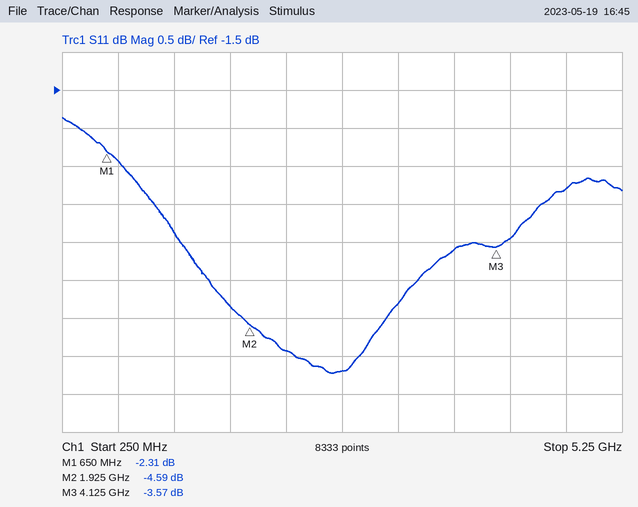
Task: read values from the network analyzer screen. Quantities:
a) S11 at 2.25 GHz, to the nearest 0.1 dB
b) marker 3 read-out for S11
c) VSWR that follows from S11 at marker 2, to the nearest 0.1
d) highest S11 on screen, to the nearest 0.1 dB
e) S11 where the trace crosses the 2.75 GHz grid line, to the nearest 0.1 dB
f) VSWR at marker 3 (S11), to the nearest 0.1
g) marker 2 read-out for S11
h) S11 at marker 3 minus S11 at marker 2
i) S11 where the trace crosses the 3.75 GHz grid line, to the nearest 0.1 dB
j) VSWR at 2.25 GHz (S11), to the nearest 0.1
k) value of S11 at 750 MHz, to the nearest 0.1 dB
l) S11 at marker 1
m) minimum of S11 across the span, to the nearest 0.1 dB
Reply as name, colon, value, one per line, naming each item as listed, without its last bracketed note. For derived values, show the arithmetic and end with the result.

S11 at 2.25 GHz, to the nearest 0.1 dB: -4.9 dB
marker 3 read-out for S11: -3.57 dB
VSWR that follows from S11 at marker 2, to the nearest 0.1: (1 + 0.5895)/(1 − 0.5895) ≈ 3.9
highest S11 on screen, to the nearest 0.1 dB: -1.9 dB
S11 where the trace crosses the 2.75 GHz grid line, to the nearest 0.1 dB: -5.2 dB
VSWR at marker 3 (S11), to the nearest 0.1: (1 + 0.6630)/(1 − 0.6630) ≈ 4.9
marker 2 read-out for S11: -4.59 dB
S11 at marker 3 minus S11 at marker 2: -3.57 − (-4.59) = 1.02 dB
S11 where the trace crosses the 3.75 GHz grid line, to the nearest 0.1 dB: -3.6 dB
VSWR at 2.25 GHz (S11), to the nearest 0.1: |Γ| = 10^(-4.9/20) = 0.5689; VSWR = (1 + 0.5689)/(1 − 0.5689) ≈ 3.6
value of S11 at 750 MHz, to the nearest 0.1 dB: -2.4 dB
S11 at marker 1: -2.31 dB
minimum of S11 across the span, to the nearest 0.1 dB: -5.2 dB
